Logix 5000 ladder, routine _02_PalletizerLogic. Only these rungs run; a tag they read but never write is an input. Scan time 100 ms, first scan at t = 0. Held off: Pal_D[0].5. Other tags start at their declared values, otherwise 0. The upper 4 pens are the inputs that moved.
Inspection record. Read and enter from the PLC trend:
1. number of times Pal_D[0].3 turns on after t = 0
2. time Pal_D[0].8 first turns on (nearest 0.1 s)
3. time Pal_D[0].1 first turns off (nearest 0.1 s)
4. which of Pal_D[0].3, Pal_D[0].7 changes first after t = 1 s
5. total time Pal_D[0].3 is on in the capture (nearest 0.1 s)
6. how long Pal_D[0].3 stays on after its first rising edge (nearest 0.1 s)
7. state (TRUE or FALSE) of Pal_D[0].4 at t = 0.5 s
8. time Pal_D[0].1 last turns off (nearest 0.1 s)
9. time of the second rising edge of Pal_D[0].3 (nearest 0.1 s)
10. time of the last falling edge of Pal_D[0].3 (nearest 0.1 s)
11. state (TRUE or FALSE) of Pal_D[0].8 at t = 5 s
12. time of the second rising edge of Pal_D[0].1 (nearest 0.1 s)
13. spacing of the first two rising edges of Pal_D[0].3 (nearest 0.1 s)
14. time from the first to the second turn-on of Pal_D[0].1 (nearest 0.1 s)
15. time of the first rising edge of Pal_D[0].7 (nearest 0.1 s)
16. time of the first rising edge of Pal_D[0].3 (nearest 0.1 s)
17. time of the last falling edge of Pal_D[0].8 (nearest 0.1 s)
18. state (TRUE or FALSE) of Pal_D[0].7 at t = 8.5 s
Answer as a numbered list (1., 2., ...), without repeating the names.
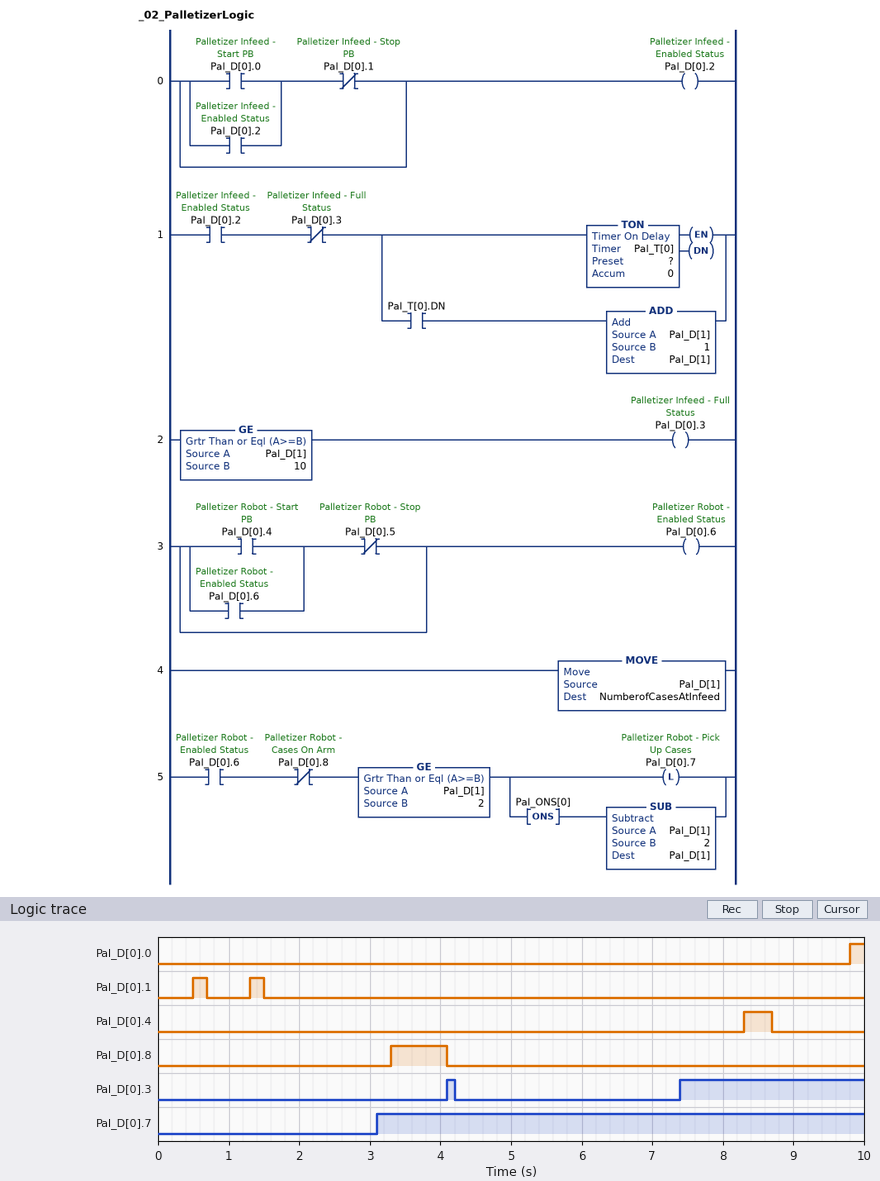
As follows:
1. 2
2. 3.3 s
3. 0.7 s
4. Pal_D[0].7
5. 2.7 s
6. 0.1 s
7. FALSE
8. 1.5 s
9. 7.4 s
10. 4.2 s
11. FALSE
12. 1.3 s
13. 3.3 s
14. 0.8 s
15. 3.1 s
16. 4.1 s
17. 4.1 s
18. TRUE
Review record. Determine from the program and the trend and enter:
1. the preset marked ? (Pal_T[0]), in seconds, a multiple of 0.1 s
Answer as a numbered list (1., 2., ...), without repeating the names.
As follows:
1. 3.0 s
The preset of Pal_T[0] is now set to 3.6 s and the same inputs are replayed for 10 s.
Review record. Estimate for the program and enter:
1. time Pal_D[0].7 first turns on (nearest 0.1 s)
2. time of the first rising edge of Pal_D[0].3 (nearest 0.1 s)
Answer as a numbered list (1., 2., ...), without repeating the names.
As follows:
1. 4.1 s
2. 4.7 s
